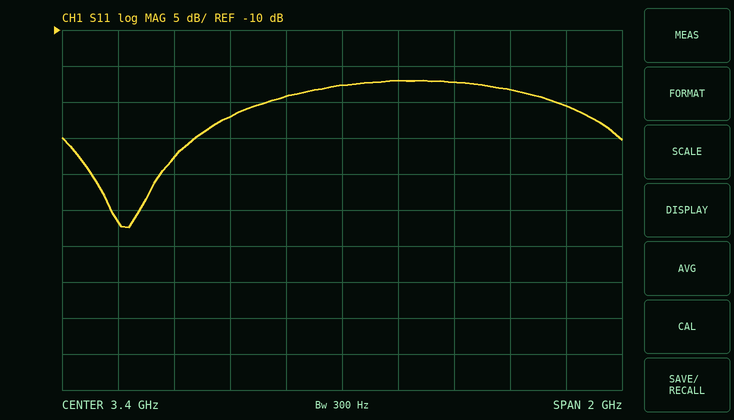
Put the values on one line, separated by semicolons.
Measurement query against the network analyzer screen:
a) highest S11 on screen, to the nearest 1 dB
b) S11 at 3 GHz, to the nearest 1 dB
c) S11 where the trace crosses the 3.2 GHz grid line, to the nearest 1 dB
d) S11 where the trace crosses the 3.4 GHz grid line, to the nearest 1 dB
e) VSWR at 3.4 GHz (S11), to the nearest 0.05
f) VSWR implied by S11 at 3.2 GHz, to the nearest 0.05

-17 dB; -22 dB; -19 dB; -18 dB; 1.30; 1.25
